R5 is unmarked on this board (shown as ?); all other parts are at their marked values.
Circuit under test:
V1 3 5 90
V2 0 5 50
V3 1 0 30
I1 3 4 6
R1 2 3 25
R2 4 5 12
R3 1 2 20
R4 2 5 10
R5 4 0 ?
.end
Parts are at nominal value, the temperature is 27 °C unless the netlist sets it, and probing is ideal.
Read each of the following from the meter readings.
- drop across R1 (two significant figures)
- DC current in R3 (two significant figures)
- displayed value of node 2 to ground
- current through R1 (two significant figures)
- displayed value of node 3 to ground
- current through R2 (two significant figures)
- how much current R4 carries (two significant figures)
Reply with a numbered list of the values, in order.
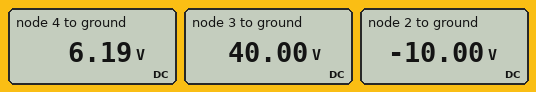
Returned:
1. 50 V
2. 2.0 A
3. -10.00 V
4. 2.0 A
5. 40.00 V
6. 4.7 A
7. 4.0 A
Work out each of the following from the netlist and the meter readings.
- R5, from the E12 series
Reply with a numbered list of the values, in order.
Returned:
1. 4.7 Ω
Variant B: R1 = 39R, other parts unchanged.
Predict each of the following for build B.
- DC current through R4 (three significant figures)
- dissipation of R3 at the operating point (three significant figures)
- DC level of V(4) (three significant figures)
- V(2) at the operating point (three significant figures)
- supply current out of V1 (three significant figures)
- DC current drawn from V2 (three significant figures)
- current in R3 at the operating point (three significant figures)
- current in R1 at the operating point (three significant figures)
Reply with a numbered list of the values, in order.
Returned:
1. 3.59 A
2. 97.2 W
3. 6.19 V
4. -14.1 V
5. 7.39 A
6. 887 mA
7. 2.20 A
8. 1.39 A
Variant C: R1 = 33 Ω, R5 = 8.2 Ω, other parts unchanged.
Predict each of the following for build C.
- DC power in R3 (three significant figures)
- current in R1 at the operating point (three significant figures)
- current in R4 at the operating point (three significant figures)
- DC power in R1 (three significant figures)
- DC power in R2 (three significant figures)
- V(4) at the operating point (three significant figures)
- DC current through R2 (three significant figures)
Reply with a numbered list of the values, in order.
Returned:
1. 91.1 W
2. 1.60 A
3. 3.73 A
4. 84.1 W
5. 289 W
6. 8.93 V
7. 4.91 A
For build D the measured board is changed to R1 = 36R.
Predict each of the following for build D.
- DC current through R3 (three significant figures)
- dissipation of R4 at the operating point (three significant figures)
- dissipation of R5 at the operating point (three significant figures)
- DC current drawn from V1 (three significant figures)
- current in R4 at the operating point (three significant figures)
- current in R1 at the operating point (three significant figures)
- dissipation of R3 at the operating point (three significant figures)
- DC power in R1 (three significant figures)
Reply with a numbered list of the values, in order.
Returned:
1. 2.17 A
2. 134 W
3. 8.16 W
4. 7.48 A
5. 3.66 A
6. 1.48 A
7. 94.3 W
8. 79.3 W
